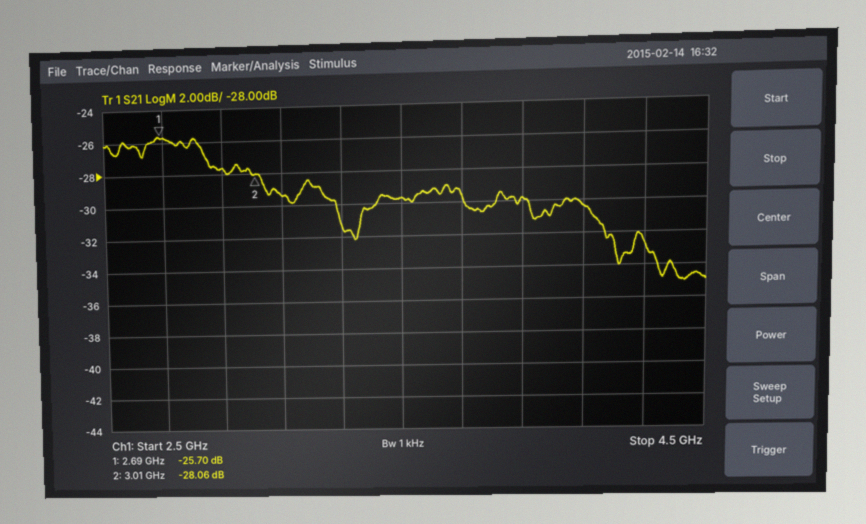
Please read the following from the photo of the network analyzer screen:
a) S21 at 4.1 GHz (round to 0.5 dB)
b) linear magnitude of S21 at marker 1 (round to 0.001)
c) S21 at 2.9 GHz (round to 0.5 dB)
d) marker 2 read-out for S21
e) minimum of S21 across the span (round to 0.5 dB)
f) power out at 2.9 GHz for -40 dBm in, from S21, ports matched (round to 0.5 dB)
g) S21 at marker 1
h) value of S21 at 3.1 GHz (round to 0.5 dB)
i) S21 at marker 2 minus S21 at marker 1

-30.5 dB
0.052
-27.5 dB
-28.06 dB
-35.0 dB
-67.5 dBm
-25.70 dB
-29.5 dB
-2.36 dB
